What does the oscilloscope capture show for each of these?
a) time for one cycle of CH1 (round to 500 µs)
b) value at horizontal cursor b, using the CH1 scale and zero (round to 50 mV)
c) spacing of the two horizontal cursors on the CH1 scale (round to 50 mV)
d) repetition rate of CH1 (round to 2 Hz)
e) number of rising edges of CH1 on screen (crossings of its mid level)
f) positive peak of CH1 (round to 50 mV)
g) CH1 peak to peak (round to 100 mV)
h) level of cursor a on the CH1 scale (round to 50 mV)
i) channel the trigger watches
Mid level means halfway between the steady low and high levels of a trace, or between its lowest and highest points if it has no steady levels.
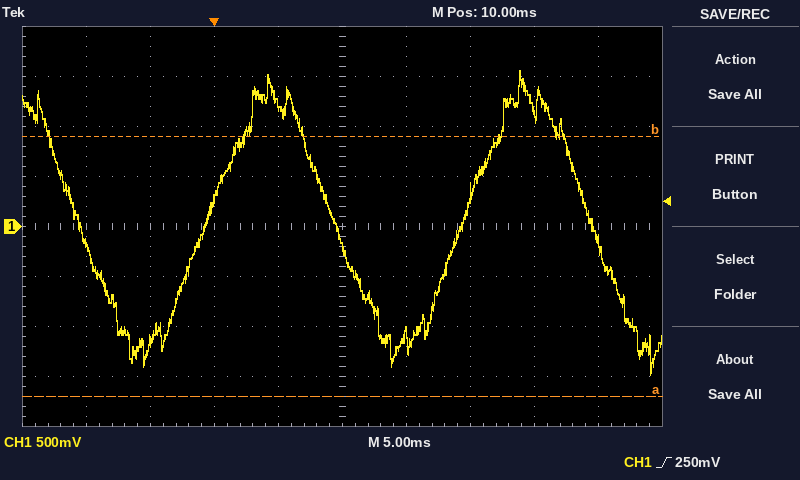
20.0 ms
900 mV
2.60 V
50 Hz
2
1.55 V
3.00 V
-1.70 V
CH1
